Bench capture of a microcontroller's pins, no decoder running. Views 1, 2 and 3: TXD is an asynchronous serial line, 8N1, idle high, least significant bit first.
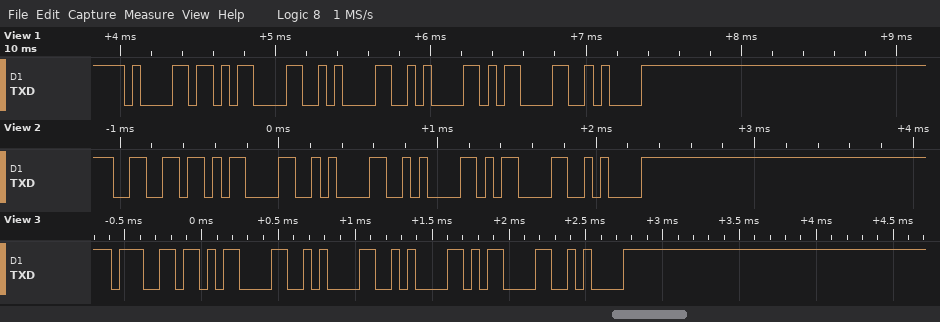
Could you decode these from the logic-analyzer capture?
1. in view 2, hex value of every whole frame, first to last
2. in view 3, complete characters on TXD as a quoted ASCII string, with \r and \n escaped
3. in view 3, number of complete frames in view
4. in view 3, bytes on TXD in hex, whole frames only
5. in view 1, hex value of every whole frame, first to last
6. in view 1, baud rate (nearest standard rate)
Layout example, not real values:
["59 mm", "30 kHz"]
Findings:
["66 0D 0A 0A 0D 0A", "\"g\\r\\n\\n\\r\\n\"", "6", "67 0D 0A 0A 0D 0A", "0x61 0x0D 0x0A 0x0A 0x0D 0x0A", "19200 baud"]
